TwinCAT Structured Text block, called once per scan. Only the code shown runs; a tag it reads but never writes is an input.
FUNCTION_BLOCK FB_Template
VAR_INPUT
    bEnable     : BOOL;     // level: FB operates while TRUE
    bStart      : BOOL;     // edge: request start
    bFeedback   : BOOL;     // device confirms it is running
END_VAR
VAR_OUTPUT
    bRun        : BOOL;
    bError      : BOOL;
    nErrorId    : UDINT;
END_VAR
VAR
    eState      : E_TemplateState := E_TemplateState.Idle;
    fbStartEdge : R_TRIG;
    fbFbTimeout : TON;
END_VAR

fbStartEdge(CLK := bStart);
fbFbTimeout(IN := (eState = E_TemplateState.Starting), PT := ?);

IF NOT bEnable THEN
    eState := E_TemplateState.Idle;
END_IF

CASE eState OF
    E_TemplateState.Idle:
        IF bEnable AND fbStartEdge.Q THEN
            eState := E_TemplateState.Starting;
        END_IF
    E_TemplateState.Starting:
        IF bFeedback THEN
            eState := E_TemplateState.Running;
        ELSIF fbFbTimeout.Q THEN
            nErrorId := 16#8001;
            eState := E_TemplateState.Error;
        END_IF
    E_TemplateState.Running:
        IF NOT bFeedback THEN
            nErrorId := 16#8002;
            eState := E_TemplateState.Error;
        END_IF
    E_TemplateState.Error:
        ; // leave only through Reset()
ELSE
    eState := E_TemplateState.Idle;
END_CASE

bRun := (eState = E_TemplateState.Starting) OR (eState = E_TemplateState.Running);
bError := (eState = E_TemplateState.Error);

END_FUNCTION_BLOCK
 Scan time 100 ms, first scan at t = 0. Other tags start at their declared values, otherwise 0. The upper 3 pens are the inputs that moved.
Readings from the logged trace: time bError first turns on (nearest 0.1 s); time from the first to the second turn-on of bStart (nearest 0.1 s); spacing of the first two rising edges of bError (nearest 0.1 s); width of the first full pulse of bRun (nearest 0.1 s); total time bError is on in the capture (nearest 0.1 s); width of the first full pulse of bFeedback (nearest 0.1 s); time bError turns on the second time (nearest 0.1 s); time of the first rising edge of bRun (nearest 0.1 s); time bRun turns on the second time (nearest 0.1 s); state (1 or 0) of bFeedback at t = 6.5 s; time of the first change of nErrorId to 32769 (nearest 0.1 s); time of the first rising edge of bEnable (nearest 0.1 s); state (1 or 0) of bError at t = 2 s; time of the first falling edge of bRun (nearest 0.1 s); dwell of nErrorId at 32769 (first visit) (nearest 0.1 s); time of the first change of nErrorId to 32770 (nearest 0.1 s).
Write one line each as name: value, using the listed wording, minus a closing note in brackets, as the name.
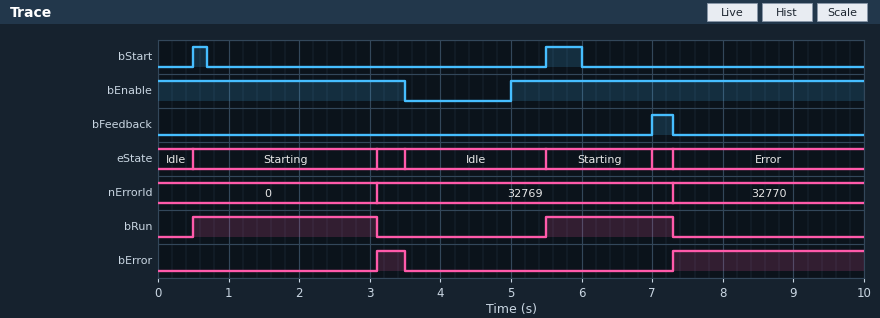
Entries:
time bError first turns on: 3.1 s
time from the first to the second turn-on of bStart: 5.0 s
spacing of the first two rising edges of bError: 4.2 s
width of the first full pulse of bRun: 2.6 s
total time bError is on in the capture: 3.1 s
width of the first full pulse of bFeedback: 0.3 s
time bError turns on the second time: 7.3 s
time of the first rising edge of bRun: 0.5 s
time bRun turns on the second time: 5.5 s
state (1 or 0) of bFeedback at t = 6.5 s: 0
time of the first change of nErrorId to 32769: 3.1 s
time of the first rising edge of bEnable: 5.0 s
state (1 or 0) of bError at t = 2 s: 0
time of the first falling edge of bRun: 3.1 s
dwell of nErrorId at 32769 (first visit): 4.2 s
time of the first change of nErrorId to 32770: 7.3 s
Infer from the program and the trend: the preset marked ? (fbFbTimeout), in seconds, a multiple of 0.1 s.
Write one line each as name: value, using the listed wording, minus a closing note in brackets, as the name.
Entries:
the preset marked ? (fbFbTimeout), in seconds, a multiple of 0.1 s: 2.5 s
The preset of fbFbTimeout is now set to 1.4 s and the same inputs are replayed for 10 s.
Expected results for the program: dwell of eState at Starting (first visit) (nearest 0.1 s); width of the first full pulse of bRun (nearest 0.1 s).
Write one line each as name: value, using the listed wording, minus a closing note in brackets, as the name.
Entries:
dwell of eState at Starting (first visit): 1.5 s
width of the first full pulse of bRun: 1.5 s
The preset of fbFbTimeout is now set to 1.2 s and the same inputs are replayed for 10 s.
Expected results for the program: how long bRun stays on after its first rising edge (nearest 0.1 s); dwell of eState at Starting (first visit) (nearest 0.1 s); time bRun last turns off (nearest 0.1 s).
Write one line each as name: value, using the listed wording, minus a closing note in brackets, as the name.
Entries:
how long bRun stays on after its first rising edge: 1.3 s
dwell of eState at Starting (first visit): 1.3 s
time bRun last turns off: 6.8 s
